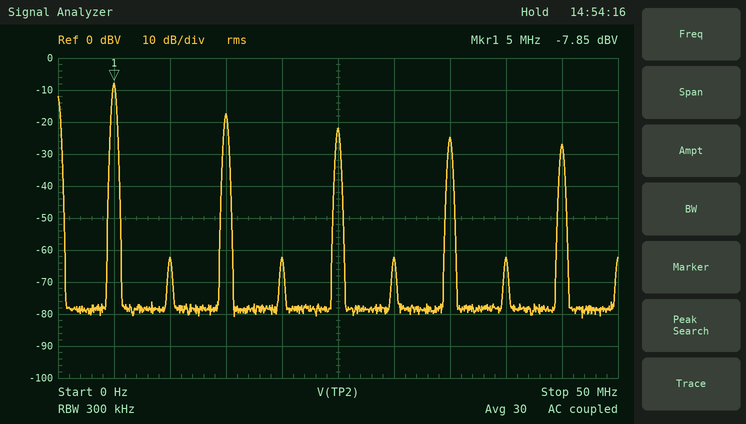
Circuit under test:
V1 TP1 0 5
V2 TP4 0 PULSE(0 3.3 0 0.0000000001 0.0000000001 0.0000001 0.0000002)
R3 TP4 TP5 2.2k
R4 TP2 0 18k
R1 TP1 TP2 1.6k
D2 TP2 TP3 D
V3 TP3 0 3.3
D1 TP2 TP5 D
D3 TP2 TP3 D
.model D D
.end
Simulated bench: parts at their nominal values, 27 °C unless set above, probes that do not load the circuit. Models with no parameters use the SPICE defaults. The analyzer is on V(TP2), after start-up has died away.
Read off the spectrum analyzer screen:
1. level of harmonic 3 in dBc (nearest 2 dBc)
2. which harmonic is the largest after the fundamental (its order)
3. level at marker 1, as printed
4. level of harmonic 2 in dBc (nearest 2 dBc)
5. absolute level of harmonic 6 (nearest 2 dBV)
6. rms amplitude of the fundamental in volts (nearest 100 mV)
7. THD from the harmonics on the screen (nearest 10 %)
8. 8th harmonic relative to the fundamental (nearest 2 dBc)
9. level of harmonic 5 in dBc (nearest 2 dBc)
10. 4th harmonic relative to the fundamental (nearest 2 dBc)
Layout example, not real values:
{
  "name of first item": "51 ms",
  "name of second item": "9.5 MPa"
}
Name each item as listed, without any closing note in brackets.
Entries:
{
  "level of harmonic 3 in dBc": "-10 dBc",
  "which harmonic is the largest after the fundamental": "3",
  "level at marker 1, as printed": "-7.85 dBV",
  "level of harmonic 2 in dBc": "-54 dBc",
  "absolute level of harmonic 6": "-62 dBV",
  "rms amplitude of the fundamental in volts": "400 mV",
  "THD from the harmonics on the screen": "40 %",
  "8th harmonic relative to the fundamental": "-54 dBc",
  "level of harmonic 5 in dBc": "-14 dBc",
  "4th harmonic relative to the fundamental": "-54 dBc"
}
